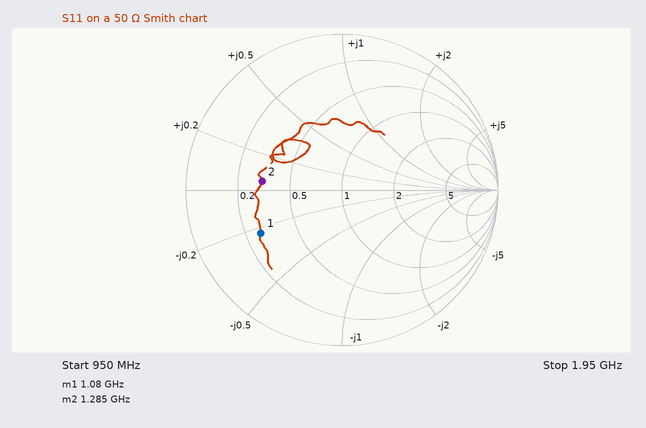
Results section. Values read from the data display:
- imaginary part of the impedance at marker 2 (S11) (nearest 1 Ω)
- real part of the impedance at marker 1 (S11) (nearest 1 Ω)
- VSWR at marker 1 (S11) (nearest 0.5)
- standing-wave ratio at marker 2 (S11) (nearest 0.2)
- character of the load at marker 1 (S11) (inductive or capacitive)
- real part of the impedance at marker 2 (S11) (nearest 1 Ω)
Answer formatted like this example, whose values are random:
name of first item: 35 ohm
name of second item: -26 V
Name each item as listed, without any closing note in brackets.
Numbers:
imaginary part of the impedance at marker 2 (S11): +2 Ω
real part of the impedance at marker 1 (S11): 14 Ω
VSWR at marker 1 (S11): 4.0
standing-wave ratio at marker 2 (S11): 3.2
character of the load at marker 1 (S11): capacitive
real part of the impedance at marker 2 (S11): 16 Ω
